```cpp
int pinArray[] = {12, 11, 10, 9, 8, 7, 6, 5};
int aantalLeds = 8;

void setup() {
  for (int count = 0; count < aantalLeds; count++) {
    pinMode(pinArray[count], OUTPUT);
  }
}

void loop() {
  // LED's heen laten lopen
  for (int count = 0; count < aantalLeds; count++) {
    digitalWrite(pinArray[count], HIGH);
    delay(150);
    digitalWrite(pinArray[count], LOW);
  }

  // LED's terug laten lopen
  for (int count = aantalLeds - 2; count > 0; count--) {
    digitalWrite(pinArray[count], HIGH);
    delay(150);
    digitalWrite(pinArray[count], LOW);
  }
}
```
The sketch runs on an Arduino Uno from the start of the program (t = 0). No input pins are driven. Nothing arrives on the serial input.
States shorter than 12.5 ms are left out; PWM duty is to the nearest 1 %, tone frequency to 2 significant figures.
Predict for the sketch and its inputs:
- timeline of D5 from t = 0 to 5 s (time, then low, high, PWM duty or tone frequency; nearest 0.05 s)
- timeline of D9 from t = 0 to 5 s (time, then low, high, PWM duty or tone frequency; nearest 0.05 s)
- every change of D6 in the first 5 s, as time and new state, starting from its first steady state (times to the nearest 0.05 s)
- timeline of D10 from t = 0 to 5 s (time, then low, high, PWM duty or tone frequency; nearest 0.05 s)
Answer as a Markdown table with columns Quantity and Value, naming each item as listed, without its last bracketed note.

| Quantity | Value |
|---|---|
| timeline of D5 from t = 0 to 5 s | 0 s low; 1.05 s high; 1.2 s low; 3.15 s high; 3.3 s low |
| timeline of D9 from t = 0 to 5 s | 0 s low; 0.45 s high; 0.6 s low; 1.65 s high; 1.8 s low; 2.55 s high; 2.7 s low; 3.75 s high; 3.9 s low; 4.65 s high; 4.8 s low |
| every change of D6 in the first 5 s, as time and new state, starting from its first steady state | 0 s low; 0.9 s high; 1.05 s low; 1.2 s high; 1.35 s low; 3 s high; 3.15 s low; 3.3 s high; 3.45 s low |
| timeline of D10 from t = 0 to 5 s | 0 s low; 0.3 s high; 0.45 s low; 1.8 s high; 1.95 s low; 2.4 s high; 2.55 s low; 3.9 s high; 4.05 s low; 4.5 s high; 4.65 s low |
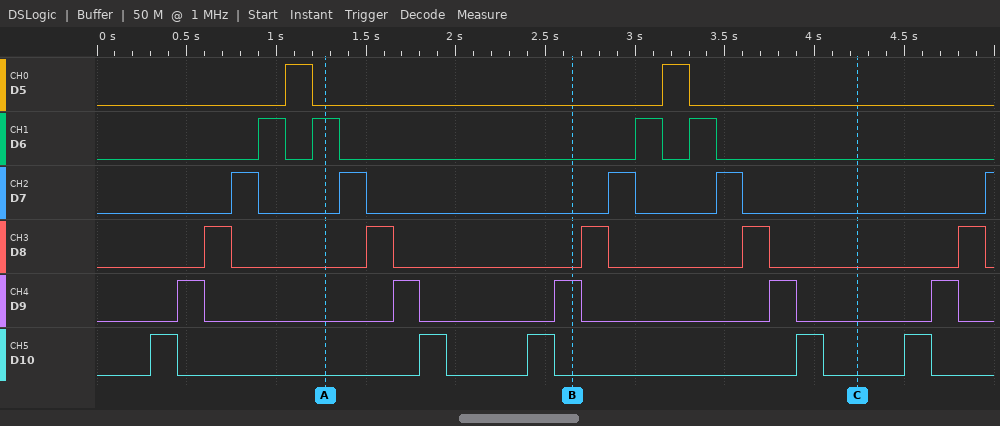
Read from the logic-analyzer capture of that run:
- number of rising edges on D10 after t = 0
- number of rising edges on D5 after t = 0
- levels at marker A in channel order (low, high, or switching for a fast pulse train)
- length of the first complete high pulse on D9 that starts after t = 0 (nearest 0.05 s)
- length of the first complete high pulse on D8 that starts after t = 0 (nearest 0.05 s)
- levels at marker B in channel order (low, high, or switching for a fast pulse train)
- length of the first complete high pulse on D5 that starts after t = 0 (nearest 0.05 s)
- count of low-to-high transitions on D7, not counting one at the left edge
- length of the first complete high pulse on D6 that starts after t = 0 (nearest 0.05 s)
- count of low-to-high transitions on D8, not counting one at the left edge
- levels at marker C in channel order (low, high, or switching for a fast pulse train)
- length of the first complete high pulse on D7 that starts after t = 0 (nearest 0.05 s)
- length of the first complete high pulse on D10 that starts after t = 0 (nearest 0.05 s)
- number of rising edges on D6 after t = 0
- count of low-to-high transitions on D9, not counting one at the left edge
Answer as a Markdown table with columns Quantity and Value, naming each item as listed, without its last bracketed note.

| Quantity | Value |
|---|---|
| number of rising edges on D10 after t = 0 | 5 |
| number of rising edges on D5 after t = 0 | 2 |
| levels at marker A in channel order | D5 low, D6 high, D7 low, D8 low, D9 low, D10 low |
| length of the first complete high pulse on D9 that starts after t = 0 | 0.15 s |
| length of the first complete high pulse on D8 that starts after t = 0 | 0.15 s |
| levels at marker B in channel order | D5 low, D6 low, D7 low, D8 low, D9 high, D10 low |
| length of the first complete high pulse on D5 that starts after t = 0 | 0.15 s |
| count of low-to-high transitions on D7, not counting one at the left edge | 5 |
| length of the first complete high pulse on D6 that starts after t = 0 | 0.15 s |
| count of low-to-high transitions on D8, not counting one at the left edge | 5 |
| levels at marker C in channel order | D5 low, D6 low, D7 low, D8 low, D9 low, D10 low |
| length of the first complete high pulse on D7 that starts after t = 0 | 0.15 s |
| length of the first complete high pulse on D10 that starts after t = 0 | 0.15 s |
| number of rising edges on D6 after t = 0 | 4 |
| count of low-to-high transitions on D9, not counting one at the left edge | 5 |
